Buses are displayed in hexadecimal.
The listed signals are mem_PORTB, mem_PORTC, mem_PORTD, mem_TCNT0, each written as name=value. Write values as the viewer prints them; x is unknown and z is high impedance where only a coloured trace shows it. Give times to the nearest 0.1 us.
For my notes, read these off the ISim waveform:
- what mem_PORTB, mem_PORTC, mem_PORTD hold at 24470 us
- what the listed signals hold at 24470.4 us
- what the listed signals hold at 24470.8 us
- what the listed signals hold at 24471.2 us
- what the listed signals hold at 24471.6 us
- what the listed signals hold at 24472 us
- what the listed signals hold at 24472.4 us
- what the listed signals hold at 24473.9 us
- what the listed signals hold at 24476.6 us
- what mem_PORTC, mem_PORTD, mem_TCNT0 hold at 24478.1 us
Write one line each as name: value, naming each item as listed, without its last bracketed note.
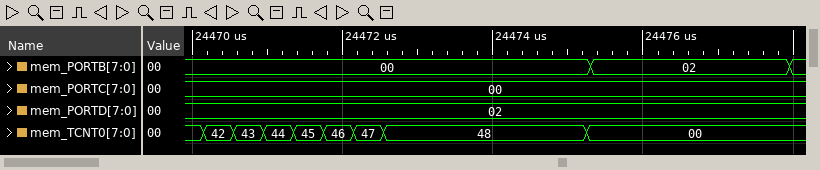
what mem_PORTB, mem_PORTC, mem_PORTD hold at 24470 us: mem_PORTB=00, mem_PORTC=00, mem_PORTD=02
what the listed signals hold at 24470.4 us: mem_PORTB=00, mem_PORTC=00, mem_PORTD=02, mem_TCNT0=42
what the listed signals hold at 24470.8 us: mem_PORTB=00, mem_PORTC=00, mem_PORTD=02, mem_TCNT0=43
what the listed signals hold at 24471.2 us: mem_PORTB=00, mem_PORTC=00, mem_PORTD=02, mem_TCNT0=44
what the listed signals hold at 24471.6 us: mem_PORTB=00, mem_PORTC=00, mem_PORTD=02, mem_TCNT0=45
what the listed signals hold at 24472 us: mem_PORTB=00, mem_PORTC=00, mem_PORTD=02, mem_TCNT0=46
what the listed signals hold at 24472.4 us: mem_PORTB=00, mem_PORTC=00, mem_PORTD=02, mem_TCNT0=47
what the listed signals hold at 24473.9 us: mem_PORTB=00, mem_PORTC=00, mem_PORTD=02, mem_TCNT0=48
what the listed signals hold at 24476.6 us: mem_PORTB=02, mem_PORTC=00, mem_PORTD=02, mem_TCNT0=00
what mem_PORTC, mem_PORTD, mem_TCNT0 hold at 24478.1 us: mem_PORTC=00, mem_PORTD=02, mem_TCNT0=00
